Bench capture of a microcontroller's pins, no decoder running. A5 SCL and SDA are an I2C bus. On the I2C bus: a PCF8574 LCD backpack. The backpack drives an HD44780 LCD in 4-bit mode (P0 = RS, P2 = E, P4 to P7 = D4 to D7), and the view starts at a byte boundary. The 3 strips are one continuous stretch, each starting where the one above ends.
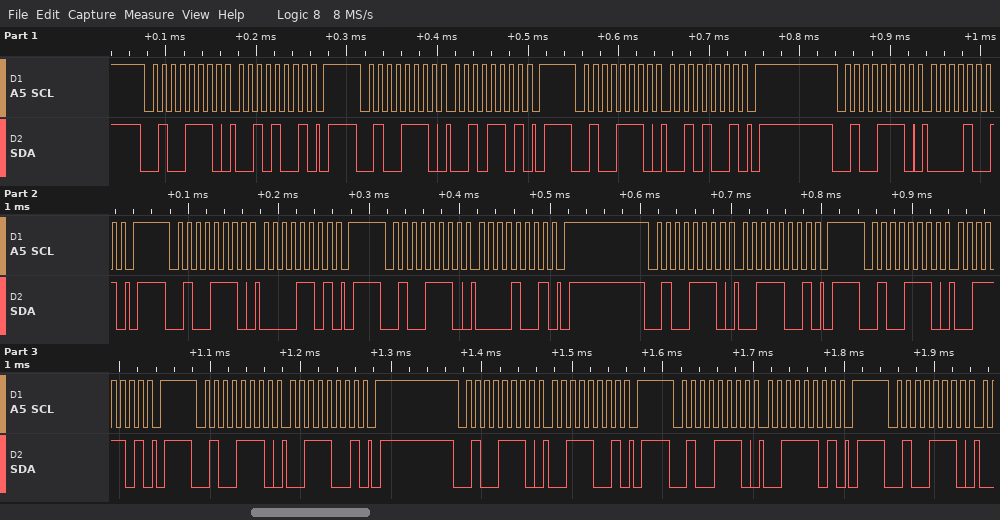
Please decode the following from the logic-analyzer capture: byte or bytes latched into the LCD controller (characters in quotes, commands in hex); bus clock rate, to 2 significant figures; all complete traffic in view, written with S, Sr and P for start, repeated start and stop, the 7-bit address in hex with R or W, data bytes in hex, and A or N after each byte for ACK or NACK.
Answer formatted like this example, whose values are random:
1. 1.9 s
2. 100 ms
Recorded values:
1. ' '
2. 100 kHz
3. S 27W A 29 A P S 27W A 2D A P S 27W A 29 A P S 27W A 09 A P S 27W A 0D A P S 27W A 09 A P S 27W A 39 A P S 27W A 3D A P S 27W A 39 A P S 27W A 39 A P S 27W A 3D A P S 27W A
